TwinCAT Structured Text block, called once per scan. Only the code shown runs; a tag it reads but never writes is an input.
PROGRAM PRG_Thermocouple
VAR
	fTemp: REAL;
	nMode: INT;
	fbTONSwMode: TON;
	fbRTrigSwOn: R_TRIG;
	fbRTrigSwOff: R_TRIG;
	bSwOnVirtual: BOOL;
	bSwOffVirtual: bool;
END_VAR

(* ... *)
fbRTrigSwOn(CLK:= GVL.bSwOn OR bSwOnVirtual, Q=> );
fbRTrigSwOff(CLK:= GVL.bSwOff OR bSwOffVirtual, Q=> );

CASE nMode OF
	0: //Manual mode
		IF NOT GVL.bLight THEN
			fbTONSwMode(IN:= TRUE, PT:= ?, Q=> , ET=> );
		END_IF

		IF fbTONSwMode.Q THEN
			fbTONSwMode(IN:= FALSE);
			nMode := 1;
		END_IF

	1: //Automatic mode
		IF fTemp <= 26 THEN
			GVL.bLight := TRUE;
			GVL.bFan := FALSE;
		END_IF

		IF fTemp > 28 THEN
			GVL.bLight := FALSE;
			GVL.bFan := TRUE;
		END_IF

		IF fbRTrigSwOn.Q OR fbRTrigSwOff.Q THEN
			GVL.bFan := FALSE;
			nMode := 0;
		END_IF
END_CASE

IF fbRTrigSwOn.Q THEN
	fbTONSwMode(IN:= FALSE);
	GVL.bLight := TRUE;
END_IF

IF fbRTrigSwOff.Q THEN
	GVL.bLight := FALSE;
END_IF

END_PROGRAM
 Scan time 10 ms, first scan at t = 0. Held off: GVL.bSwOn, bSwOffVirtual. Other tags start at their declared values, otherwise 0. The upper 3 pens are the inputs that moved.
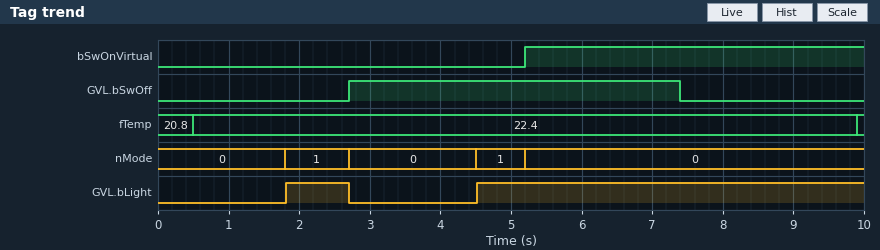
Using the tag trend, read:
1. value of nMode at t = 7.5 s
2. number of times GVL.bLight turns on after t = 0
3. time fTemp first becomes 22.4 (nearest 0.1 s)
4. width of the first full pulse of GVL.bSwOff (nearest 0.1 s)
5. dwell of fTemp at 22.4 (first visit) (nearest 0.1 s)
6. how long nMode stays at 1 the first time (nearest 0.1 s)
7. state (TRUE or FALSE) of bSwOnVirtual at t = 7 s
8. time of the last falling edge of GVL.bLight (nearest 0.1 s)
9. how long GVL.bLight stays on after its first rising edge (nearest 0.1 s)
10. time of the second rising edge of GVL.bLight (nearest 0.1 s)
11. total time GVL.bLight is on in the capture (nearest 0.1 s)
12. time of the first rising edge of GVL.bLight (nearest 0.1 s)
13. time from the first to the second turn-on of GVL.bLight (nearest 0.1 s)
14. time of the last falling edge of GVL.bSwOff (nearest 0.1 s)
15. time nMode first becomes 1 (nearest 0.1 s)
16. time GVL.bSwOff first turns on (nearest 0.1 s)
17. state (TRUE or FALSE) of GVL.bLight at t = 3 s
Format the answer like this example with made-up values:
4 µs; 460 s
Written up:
0; 2; 0.5 s; 4.7 s; 9.4 s; 0.9 s; TRUE; 2.7 s; 0.9 s; 4.5 s; 6.4 s; 1.8 s; 2.7 s; 7.4 s; 1.8 s; 2.7 s; FALSE
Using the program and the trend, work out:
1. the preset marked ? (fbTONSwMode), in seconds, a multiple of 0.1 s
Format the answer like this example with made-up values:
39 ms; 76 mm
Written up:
1.8 s
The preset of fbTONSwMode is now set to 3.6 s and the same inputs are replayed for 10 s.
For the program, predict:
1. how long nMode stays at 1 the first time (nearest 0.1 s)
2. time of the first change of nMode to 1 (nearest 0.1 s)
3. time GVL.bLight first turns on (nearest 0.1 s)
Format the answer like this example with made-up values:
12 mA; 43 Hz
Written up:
1.6 s; 3.6 s; 3.6 s
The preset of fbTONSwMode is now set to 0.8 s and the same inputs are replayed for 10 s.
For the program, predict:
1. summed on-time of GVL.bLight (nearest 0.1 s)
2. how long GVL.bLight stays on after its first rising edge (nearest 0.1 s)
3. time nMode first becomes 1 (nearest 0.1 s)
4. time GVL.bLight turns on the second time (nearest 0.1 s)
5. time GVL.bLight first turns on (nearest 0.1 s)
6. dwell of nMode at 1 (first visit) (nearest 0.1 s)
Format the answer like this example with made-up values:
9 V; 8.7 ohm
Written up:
8.4 s; 1.9 s; 0.8 s; 3.5 s; 0.8 s; 1.9 s
